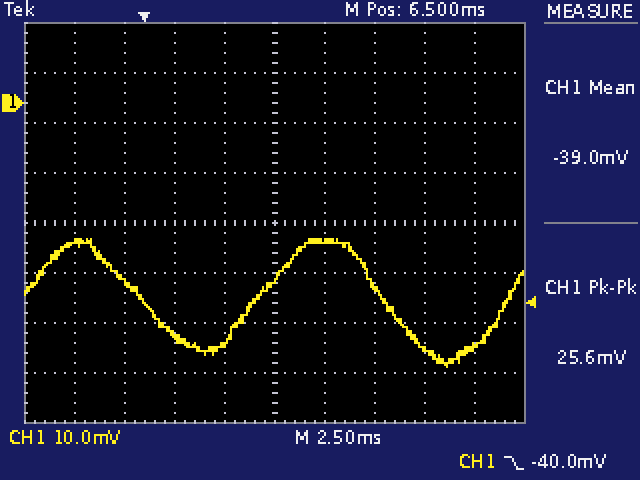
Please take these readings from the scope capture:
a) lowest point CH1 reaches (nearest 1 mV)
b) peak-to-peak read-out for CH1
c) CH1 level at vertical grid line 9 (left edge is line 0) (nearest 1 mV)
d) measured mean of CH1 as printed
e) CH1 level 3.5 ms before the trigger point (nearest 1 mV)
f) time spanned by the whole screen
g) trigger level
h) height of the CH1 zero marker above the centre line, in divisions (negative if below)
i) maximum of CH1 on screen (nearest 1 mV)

-53 mV
25.6 mV
-49 mV
-39.0 mV
-28 mV
25 ms
-40.0 mV
+2.4 div
-27 mV
